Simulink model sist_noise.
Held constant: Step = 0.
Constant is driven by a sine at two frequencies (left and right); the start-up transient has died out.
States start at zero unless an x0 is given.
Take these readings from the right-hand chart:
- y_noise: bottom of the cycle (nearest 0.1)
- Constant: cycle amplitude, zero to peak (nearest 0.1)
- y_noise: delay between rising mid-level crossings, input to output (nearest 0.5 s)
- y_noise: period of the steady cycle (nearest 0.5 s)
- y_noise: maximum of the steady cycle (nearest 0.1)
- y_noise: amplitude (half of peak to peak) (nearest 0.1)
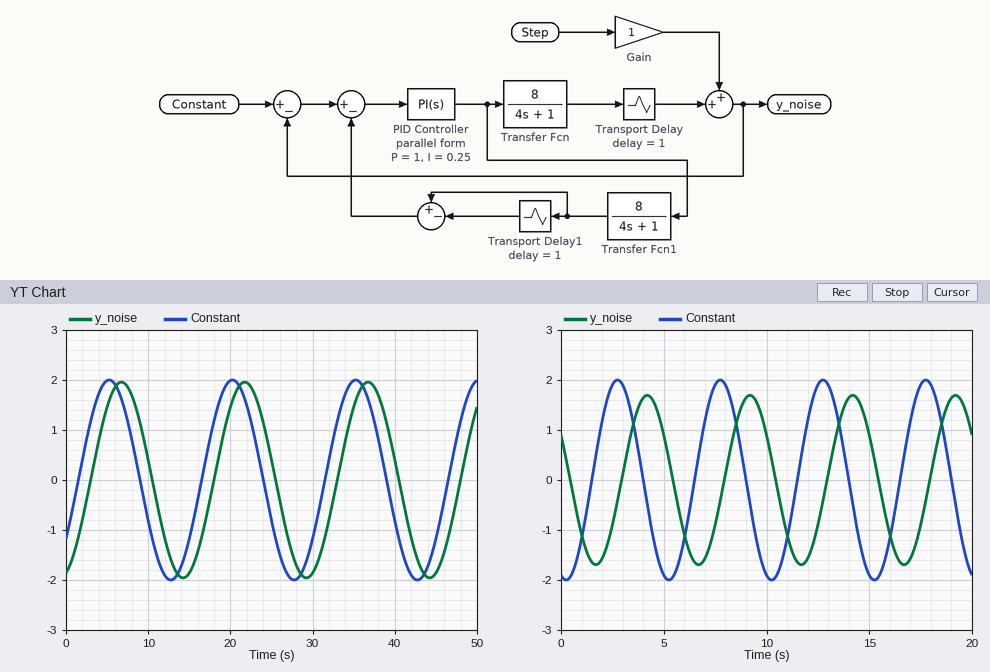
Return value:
-1.7
2.0
1.5 s
5.0 s
1.7
1.7
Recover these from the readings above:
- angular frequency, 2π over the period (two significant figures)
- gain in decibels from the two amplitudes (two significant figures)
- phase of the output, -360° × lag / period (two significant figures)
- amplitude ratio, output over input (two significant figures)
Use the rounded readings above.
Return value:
1.3 rad/s
-1.4 dB
-110°
0.85
